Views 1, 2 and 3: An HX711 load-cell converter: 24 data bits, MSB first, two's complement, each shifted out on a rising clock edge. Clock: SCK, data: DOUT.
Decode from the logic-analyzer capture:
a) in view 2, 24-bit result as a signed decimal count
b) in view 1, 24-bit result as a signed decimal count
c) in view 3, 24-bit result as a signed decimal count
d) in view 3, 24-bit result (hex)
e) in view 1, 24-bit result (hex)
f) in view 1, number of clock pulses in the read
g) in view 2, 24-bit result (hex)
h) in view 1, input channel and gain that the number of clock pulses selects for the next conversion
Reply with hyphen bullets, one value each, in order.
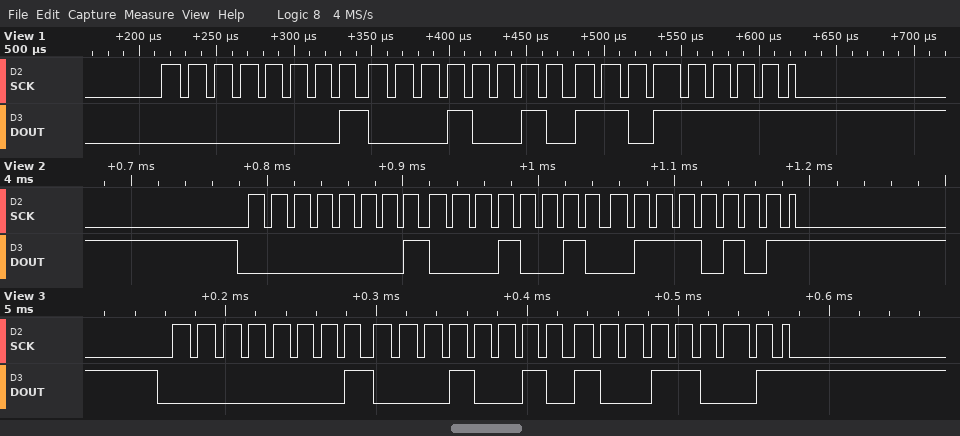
- 70261
- 70367
- 70297
- 0x011299
- 0x0112DF
- 25
- 0x011275
- channel A, gain 128
